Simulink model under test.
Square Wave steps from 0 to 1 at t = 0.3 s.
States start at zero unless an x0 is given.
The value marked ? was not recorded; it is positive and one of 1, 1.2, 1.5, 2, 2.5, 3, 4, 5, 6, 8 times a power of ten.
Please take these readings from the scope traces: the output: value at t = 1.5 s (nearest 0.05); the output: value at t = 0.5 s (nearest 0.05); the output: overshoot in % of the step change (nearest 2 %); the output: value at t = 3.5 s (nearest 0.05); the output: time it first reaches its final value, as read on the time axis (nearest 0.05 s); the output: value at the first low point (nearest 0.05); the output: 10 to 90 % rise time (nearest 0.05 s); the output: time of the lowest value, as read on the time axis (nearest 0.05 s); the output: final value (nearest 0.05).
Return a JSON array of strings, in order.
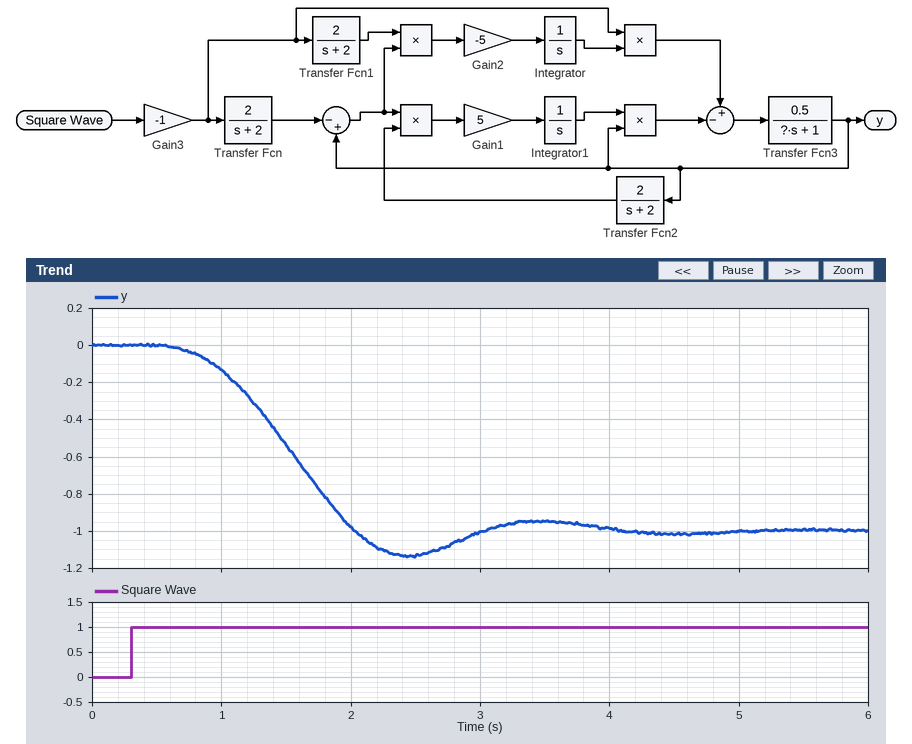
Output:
["-0.55", "0.00", "14 %", "-0.95", "2.05 s", "-1.15", "0.95 s", "2.45 s", "-1.00"]
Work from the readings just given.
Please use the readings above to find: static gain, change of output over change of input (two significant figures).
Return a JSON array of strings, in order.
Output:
["-1.0"]
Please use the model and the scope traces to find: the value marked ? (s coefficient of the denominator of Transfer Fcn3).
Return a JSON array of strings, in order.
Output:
["0.5"]
